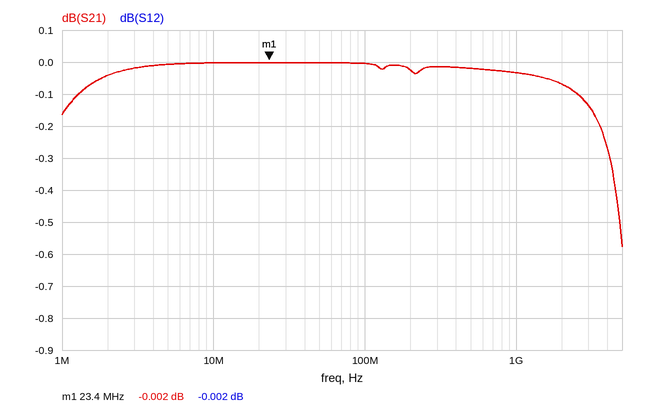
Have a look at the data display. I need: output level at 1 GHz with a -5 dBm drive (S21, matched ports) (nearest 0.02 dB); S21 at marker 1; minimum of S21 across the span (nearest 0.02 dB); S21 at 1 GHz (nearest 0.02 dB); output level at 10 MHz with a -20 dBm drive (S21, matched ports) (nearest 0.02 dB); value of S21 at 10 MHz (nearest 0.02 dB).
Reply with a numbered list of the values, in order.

1. -5.04 dBm
2. -0.002 dB
3. -0.58 dB
4. -0.04 dB
5. -20.00 dBm
6. 0.00 dB
